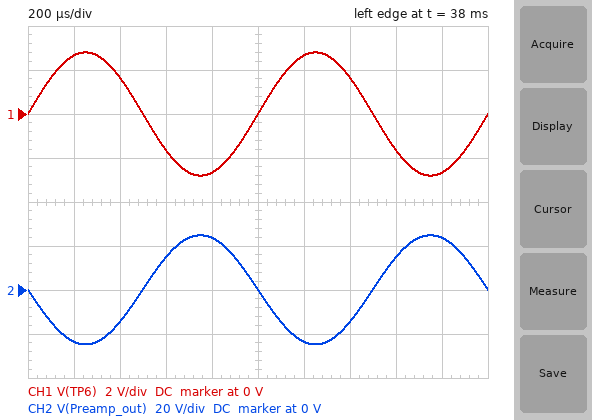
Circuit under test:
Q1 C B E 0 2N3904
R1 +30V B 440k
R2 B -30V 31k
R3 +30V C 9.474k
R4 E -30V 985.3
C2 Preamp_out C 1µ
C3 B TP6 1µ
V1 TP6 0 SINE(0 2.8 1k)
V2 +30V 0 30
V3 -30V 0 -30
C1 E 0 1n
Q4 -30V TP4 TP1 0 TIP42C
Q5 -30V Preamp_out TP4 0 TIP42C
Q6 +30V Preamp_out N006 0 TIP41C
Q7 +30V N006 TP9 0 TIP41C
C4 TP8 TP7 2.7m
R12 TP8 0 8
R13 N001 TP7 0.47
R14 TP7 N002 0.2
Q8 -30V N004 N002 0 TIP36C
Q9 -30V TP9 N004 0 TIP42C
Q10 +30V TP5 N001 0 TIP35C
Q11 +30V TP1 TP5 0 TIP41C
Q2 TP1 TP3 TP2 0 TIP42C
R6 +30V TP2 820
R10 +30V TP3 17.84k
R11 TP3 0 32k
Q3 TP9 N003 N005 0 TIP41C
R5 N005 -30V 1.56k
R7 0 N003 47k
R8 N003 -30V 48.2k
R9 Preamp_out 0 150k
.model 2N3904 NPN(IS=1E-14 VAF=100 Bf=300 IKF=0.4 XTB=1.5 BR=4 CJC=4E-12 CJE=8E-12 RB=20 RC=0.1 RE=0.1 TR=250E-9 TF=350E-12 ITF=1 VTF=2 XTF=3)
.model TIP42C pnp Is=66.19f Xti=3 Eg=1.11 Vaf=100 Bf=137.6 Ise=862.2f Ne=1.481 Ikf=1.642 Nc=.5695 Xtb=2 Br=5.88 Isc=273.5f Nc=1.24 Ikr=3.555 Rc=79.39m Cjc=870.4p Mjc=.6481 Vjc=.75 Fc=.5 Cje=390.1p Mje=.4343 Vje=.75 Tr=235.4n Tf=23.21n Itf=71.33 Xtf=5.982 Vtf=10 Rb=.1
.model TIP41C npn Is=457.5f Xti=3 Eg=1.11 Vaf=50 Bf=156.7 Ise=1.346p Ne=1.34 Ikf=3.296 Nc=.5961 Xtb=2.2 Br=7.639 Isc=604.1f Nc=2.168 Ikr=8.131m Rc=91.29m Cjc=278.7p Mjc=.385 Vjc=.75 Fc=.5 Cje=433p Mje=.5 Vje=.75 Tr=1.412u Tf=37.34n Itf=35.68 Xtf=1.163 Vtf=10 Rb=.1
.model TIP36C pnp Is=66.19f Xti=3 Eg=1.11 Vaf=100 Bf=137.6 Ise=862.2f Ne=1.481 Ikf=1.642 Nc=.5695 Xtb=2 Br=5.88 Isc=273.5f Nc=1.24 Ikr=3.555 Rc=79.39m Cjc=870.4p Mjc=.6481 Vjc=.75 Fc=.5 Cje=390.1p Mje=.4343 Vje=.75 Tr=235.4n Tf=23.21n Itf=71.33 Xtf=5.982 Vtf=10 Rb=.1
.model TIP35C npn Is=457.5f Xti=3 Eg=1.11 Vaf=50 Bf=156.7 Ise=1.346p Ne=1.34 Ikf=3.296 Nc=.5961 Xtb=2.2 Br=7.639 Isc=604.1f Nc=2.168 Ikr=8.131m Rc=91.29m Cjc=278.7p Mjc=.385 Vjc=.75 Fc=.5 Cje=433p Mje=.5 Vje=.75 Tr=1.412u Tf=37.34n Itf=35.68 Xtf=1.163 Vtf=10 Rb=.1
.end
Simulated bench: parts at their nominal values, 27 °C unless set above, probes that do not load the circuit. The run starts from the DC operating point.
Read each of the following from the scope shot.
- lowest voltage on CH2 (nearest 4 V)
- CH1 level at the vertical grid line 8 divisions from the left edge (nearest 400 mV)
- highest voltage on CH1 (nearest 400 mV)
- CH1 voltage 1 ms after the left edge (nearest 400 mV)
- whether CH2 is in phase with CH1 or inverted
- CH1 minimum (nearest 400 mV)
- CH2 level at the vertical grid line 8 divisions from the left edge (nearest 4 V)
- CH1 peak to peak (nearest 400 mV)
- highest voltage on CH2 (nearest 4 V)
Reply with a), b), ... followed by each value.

a) -24 V
b) -1.6 V
c) 2.8 V
d) 0 V
e) inverted
f) -2.8 V
g) 16 V
h) 5.6 V
i) 24 V
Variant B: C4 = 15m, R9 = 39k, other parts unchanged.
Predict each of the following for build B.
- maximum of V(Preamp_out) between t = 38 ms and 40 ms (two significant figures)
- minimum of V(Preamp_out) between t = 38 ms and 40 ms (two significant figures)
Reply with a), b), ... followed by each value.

a) 21 V
b) -21 V
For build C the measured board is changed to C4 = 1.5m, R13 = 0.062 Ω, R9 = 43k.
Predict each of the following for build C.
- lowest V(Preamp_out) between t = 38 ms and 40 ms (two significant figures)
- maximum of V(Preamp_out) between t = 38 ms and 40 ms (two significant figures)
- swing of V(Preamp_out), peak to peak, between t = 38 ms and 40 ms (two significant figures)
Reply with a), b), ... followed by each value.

a) -22 V
b) 22 V
c) 43 V
